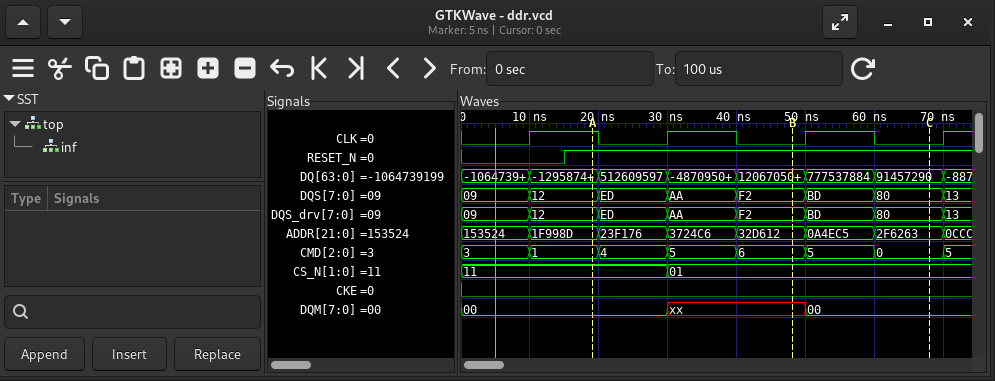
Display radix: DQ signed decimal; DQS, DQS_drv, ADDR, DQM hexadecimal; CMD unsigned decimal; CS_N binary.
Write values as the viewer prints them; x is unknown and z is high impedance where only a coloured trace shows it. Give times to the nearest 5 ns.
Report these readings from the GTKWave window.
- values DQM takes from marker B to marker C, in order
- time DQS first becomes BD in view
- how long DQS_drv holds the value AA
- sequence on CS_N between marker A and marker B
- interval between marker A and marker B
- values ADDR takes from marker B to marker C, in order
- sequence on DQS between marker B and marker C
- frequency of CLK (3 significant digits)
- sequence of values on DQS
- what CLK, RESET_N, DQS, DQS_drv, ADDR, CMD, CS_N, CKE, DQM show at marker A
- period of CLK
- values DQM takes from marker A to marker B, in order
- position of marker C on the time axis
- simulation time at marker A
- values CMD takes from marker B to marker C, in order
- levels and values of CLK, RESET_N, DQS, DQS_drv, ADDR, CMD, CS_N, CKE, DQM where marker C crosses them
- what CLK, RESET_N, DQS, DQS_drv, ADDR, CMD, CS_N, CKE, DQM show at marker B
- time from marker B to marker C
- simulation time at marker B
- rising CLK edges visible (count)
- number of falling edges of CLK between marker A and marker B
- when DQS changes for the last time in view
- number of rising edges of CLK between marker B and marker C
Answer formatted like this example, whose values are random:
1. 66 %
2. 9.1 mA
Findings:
1. xx, 00
2. 50 ns
3. 10 ns
4. 11, 01
5. 30 ns
6. 32D612, 0A4EC5, 2F6263
7. F2, BD, 80
8. 50.0 MHz
9. 09, 12, ED, AA, F2, BD, 80, 13
10. CLK=1, RESET_N=1, DQS=12, DQS_drv=12, ADDR=1F998D, CMD=1, CS_N=11, CKE=0, DQM=00
11. 20 ns
12. 00, xx
13. 70 ns
14. 20 ns
15. 6, 5, 0
16. CLK=0, RESET_N=1, DQS=80, DQS_drv=80, ADDR=2F6263, CMD=0, CS_N=01, CKE=0, DQM=00
17. CLK=0, RESET_N=1, DQS=F2, DQS_drv=F2, ADDR=32D612, CMD=6, CS_N=01, CKE=0, DQM=xx
18. 20 ns
19. 50 ns
20. 4
21. 2
22. 70 ns
23. 1
